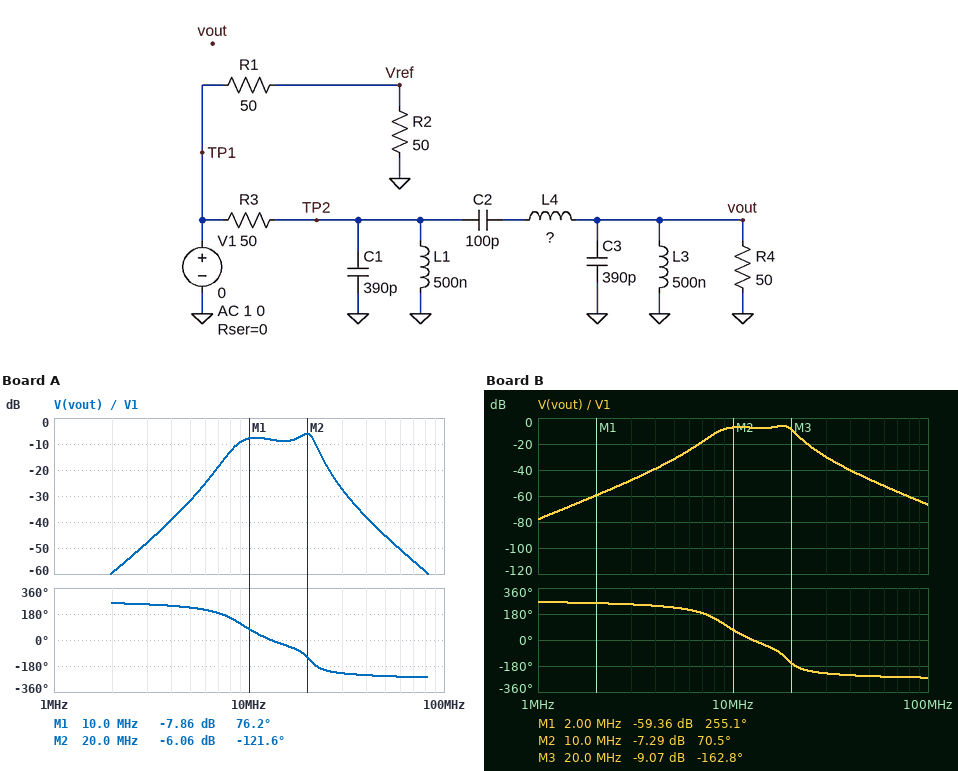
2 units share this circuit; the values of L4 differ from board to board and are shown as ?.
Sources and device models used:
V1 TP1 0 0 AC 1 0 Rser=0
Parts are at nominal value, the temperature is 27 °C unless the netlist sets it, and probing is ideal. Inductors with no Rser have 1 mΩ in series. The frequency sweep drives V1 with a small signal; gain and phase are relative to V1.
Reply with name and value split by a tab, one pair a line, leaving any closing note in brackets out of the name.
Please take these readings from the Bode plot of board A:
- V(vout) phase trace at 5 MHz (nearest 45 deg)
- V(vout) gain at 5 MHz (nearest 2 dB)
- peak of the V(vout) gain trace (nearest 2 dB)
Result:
V(vout) phase trace at 5 MHz	225 deg
V(vout) gain at 5 MHz	-32 dB
peak of the V(vout) gain trace	-6 dB
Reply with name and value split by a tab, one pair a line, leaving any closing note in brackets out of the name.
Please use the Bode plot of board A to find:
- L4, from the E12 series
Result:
L4, from the E12 series	1 µH
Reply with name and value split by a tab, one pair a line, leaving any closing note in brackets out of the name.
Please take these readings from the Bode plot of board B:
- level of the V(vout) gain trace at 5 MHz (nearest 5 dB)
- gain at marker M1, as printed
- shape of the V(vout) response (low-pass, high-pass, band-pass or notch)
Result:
level of the V(vout) gain trace at 5 MHz	-30 dB
gain at marker M1, as printed	-59.36 dB
shape of the V(vout) response	band-pass
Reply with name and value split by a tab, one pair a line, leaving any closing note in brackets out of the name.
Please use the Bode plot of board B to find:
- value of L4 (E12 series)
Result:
value of L4	1.2 µH
